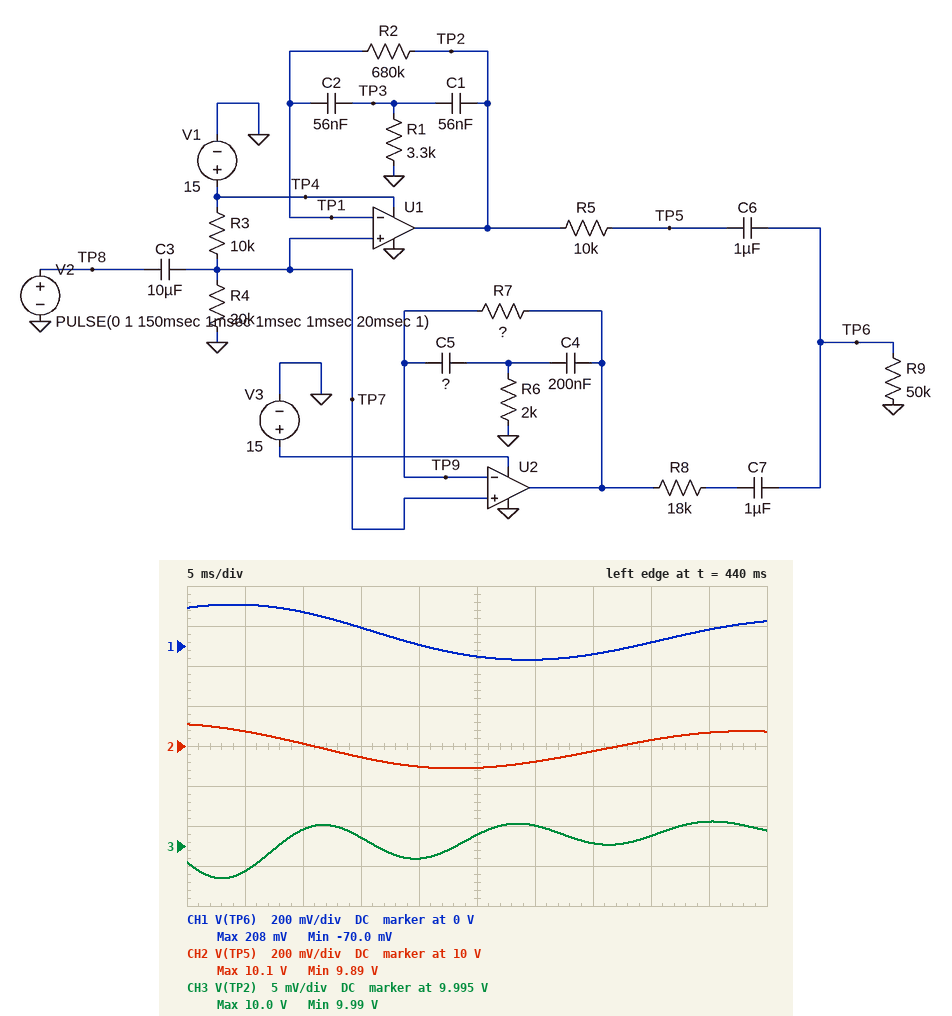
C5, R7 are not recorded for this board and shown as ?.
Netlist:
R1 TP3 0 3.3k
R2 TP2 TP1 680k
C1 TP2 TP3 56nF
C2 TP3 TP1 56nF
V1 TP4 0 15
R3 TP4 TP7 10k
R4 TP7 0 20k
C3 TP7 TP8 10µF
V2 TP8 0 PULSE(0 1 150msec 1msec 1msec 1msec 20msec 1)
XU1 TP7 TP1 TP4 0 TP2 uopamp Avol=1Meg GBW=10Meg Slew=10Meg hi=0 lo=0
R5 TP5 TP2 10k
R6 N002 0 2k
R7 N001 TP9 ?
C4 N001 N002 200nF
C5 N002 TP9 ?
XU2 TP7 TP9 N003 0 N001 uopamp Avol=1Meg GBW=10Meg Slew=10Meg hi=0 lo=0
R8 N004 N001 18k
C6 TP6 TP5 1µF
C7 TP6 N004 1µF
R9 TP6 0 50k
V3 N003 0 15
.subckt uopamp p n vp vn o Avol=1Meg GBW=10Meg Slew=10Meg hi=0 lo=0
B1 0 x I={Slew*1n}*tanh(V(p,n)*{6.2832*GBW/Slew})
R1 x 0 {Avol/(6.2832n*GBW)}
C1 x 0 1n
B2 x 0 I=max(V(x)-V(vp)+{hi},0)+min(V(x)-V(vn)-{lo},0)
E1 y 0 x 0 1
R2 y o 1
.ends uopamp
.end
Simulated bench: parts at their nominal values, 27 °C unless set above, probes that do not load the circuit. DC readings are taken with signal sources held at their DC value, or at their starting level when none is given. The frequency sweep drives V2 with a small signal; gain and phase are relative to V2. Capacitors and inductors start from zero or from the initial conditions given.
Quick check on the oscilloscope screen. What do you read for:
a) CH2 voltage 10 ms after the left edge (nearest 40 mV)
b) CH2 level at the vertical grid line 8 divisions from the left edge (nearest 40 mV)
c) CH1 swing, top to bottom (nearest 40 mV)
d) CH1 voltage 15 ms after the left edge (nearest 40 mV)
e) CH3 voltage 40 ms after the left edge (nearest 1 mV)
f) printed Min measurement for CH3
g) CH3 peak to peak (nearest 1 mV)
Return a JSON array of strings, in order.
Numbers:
["10.00 V", "10.04 V", "280 mV", "80 mV", "9.996 V", "9.99 V", "7 mV"]
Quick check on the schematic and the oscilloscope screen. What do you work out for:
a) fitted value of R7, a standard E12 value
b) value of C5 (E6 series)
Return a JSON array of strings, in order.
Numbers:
["470 kΩ", "330 nF"]
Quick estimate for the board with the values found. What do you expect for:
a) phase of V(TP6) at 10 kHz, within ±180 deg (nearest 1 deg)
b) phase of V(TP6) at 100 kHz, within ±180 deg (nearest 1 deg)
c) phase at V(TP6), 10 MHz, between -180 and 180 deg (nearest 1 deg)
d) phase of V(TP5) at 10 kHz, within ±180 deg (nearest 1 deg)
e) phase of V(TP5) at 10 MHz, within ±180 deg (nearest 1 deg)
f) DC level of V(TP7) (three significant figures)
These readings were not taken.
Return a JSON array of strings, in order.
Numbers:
["-4 deg", "-1 deg", "-45 deg", "-4 deg", "-45 deg", "10.0 V"]
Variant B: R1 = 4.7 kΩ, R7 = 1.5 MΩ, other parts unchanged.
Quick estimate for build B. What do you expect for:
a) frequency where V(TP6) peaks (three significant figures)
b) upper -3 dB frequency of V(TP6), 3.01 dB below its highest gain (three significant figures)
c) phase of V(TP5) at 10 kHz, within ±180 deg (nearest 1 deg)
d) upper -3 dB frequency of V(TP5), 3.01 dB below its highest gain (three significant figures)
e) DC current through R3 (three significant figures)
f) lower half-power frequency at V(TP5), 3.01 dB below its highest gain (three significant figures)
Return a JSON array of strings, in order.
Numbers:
["11.3 Hz", "11.7 Hz", "-3 deg", "11.8 Hz", "500 µA", "10.9 Hz"]
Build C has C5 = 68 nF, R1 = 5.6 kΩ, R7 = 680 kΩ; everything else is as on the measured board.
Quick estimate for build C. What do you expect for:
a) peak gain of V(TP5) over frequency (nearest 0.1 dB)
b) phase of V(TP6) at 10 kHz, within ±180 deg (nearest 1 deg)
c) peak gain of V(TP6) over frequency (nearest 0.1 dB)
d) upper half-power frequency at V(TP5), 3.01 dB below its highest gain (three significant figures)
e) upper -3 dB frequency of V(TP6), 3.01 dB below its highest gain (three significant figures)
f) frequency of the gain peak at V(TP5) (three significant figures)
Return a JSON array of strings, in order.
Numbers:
["32.5 dB", "-3 deg", "31.4 dB", "50.8 Hz", "51.5 Hz", "46.2 Hz"]
